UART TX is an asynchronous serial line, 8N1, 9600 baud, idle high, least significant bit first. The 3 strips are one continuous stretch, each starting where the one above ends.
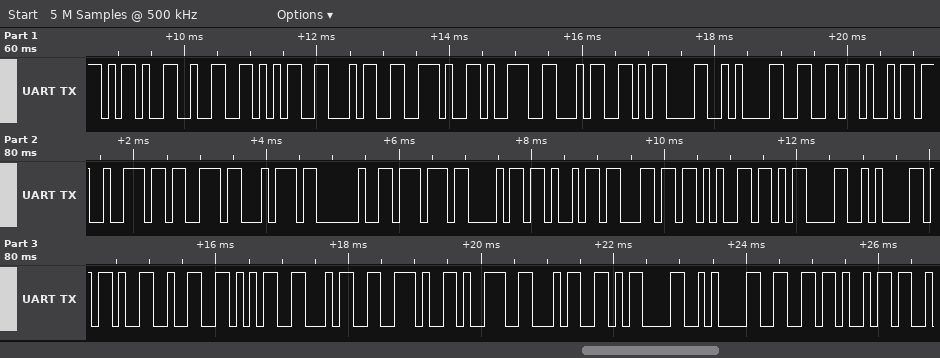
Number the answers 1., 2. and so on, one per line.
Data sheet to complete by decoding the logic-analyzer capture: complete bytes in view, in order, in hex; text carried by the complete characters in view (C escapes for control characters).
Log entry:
1. 2D 32 35 34 2E 39 34 0D 0A 66 69 72 73 74 20 77 68 69 6C 65 0D 0A 2D 32 35 34 2E 39 34 0D 0A 66 69
2. "-254.94\r\nfirst while\r\n-254.94\r\nfi"
